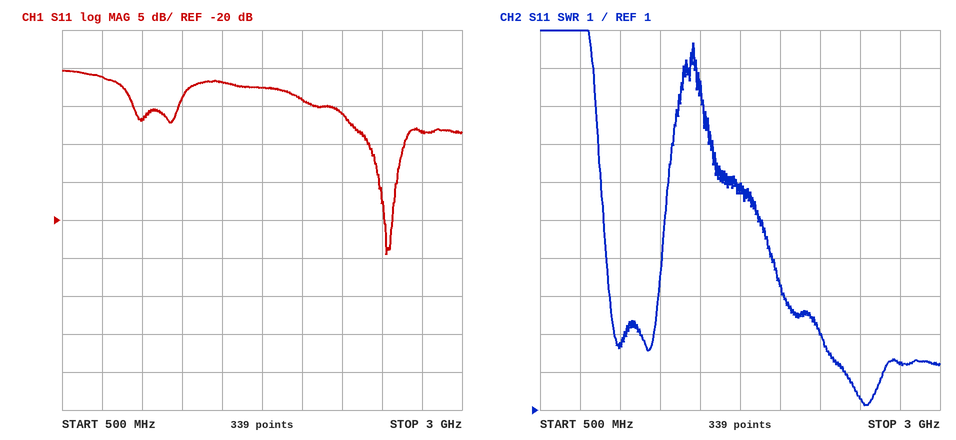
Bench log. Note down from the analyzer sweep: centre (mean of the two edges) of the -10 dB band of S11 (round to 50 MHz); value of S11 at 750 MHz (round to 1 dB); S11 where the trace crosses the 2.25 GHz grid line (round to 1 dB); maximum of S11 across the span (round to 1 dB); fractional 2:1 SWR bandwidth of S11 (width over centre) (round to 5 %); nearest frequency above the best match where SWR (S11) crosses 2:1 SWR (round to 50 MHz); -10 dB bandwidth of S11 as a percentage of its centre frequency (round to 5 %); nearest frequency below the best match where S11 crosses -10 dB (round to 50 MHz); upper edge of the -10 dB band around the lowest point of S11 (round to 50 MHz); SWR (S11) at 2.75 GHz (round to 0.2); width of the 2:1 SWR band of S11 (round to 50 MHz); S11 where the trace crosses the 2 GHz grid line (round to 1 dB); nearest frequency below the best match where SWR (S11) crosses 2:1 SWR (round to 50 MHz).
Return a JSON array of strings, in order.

["2.55 GHz", "-1 dB", "-6 dB", "0 dB", "10 %", "2.65 GHz", "10 %", "2.40 GHz", "2.65 GHz", "2.2", "250 MHz", "-4 dB", "2.40 GHz"]
